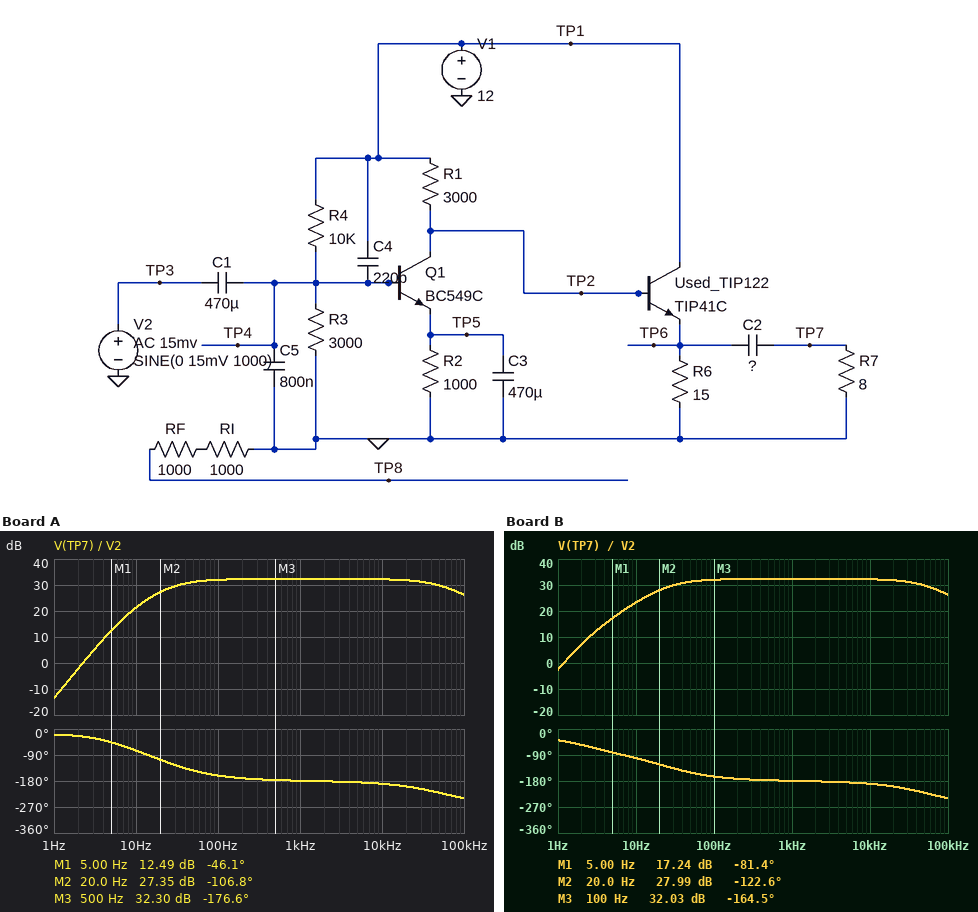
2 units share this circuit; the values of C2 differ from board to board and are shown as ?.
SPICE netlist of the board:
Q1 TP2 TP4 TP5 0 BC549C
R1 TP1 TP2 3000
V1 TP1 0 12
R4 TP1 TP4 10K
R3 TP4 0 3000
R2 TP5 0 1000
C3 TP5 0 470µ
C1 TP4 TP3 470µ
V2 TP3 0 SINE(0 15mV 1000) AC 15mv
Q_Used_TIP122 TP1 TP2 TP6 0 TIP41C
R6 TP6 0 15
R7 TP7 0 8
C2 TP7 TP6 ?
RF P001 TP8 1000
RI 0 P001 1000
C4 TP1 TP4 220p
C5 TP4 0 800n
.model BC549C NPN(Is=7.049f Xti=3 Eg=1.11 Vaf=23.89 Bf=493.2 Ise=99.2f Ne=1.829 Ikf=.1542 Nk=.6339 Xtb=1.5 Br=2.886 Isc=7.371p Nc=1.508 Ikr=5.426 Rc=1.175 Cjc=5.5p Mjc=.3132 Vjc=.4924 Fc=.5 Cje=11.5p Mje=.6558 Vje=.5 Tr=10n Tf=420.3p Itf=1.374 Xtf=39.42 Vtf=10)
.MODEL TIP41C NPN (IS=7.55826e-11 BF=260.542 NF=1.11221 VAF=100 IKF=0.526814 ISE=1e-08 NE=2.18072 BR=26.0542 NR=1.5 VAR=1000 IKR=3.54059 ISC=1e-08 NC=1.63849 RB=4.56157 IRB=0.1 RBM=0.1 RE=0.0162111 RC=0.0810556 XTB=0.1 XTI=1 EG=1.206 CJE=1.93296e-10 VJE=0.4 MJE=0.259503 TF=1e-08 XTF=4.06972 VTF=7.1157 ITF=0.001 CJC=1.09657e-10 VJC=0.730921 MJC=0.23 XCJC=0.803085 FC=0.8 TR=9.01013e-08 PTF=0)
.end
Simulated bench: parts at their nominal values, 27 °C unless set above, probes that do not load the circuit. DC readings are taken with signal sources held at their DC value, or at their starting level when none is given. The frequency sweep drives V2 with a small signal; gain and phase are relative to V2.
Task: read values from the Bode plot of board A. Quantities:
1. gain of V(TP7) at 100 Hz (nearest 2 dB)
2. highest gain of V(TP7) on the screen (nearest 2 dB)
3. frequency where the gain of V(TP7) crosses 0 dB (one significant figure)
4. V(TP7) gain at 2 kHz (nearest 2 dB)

32 dB
32 dB
2 Hz
32 dB
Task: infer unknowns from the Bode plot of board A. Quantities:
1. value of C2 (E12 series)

1.2 mF
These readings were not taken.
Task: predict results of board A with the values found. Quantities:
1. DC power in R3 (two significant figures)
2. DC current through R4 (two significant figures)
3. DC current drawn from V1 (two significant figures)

2.5 mW
920 µA
130 mA
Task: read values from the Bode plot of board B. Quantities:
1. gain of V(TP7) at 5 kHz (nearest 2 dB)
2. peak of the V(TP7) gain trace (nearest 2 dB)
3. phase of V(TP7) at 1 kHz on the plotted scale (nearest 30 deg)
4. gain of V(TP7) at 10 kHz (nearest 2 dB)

32 dB
32 dB
-180 deg
32 dB
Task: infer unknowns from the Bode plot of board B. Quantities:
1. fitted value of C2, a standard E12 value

4.7 mF
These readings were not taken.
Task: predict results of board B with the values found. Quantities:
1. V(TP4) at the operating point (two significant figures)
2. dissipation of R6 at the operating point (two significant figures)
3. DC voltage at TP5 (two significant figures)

2.8 V
250 mW
2.1 V
